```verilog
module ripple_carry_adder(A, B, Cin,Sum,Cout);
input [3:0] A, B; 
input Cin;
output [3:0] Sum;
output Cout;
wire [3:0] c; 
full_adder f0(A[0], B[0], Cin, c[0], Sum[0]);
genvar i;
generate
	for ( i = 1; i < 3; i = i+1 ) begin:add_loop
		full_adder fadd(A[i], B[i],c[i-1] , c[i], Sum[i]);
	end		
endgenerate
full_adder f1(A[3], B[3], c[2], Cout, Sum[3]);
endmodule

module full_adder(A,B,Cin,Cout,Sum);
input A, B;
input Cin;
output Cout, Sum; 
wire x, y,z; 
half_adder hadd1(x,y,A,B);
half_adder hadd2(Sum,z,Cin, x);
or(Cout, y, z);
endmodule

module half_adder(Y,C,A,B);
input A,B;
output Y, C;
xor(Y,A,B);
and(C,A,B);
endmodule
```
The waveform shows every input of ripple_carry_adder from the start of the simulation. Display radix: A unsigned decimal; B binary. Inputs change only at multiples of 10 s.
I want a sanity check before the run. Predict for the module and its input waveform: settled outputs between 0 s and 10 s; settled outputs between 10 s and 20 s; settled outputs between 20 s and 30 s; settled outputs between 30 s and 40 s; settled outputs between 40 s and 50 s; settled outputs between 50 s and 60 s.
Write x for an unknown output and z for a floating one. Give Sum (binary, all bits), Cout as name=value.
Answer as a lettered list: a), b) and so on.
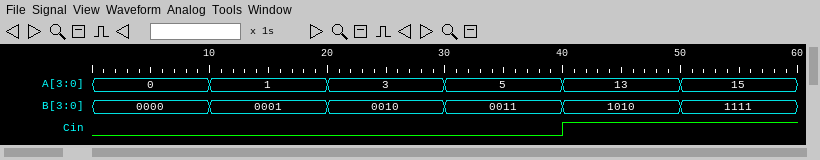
a) Sum=0000, Cout=0
b) Sum=0010, Cout=0
c) Sum=0101, Cout=0
d) Sum=1000, Cout=0
e) Sum=1000, Cout=1
f) Sum=1111, Cout=1
